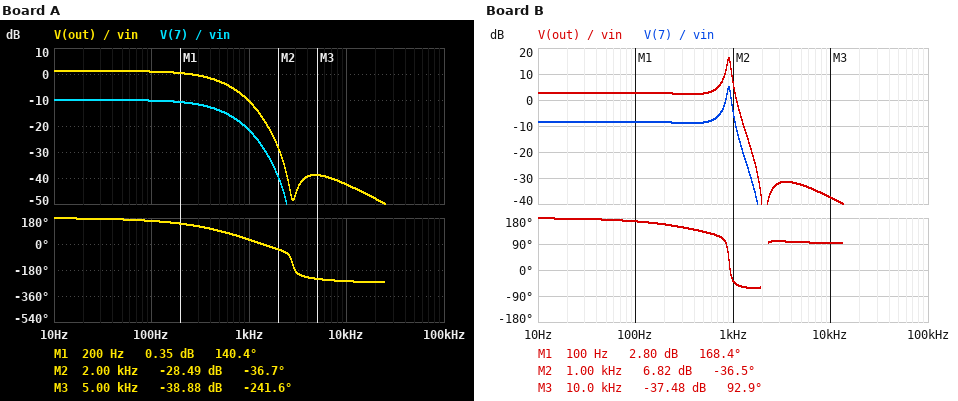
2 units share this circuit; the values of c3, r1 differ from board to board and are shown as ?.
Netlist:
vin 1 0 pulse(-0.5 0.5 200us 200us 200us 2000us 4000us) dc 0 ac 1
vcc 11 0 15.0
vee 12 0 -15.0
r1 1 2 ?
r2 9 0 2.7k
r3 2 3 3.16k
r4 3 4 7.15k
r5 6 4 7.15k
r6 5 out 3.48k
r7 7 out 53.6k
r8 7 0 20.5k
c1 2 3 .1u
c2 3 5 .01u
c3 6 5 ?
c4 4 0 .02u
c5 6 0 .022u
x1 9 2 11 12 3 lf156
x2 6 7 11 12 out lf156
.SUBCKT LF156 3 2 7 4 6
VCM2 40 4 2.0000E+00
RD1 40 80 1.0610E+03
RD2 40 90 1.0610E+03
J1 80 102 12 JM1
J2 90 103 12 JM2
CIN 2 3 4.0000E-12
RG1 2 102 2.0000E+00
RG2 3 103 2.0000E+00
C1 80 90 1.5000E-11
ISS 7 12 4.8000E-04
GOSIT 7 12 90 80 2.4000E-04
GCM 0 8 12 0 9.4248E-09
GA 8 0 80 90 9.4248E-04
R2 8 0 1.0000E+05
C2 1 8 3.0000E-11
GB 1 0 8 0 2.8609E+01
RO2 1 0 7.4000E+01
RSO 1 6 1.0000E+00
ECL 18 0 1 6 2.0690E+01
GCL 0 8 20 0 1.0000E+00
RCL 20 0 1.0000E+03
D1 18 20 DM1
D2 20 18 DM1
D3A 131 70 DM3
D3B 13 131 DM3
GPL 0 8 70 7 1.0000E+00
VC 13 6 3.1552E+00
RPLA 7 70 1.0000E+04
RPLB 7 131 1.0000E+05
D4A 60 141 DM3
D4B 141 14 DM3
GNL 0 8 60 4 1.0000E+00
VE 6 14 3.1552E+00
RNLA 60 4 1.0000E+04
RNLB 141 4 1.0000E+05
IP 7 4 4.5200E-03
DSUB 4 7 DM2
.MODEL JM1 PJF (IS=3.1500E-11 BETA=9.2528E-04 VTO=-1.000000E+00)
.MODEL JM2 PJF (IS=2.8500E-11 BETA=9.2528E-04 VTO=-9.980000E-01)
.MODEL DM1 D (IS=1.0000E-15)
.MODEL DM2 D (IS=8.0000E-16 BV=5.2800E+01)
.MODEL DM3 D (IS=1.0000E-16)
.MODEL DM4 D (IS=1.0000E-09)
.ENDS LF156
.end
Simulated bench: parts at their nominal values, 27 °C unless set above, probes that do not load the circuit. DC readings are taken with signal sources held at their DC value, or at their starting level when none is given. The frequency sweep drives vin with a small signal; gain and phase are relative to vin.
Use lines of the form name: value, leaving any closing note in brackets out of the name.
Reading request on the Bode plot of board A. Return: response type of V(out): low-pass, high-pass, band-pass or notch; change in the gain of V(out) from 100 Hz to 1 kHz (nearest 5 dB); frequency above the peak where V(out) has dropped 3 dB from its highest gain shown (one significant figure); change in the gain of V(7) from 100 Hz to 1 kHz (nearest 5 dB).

response type of V(out): low-pass, high-pass, band-pass or notch: low-pass
change in the gain of V(out) from 100 Hz to 1 kHz: -10 dB
frequency above the peak where V(out) has dropped 3 dB from its highest gain shown: 400 Hz
change in the gain of V(7) from 100 Hz to 1 kHz: -10 dB
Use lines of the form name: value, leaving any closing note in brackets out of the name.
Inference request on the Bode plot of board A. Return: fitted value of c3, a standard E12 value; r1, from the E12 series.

fitted value of c3, a standard E12 value: 5.6 nF
r1, from the E12 series: 10 kΩ
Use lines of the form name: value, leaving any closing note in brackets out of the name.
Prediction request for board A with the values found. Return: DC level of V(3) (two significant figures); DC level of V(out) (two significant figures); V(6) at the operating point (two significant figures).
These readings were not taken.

DC level of V(3): 2.6 mV
DC level of V(out): 17 mV
V(6) at the operating point: 2.6 mV
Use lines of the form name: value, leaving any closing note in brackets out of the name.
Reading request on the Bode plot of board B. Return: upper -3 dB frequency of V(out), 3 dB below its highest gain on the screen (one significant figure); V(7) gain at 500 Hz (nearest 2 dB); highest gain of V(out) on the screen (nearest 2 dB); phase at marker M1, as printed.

upper -3 dB frequency of V(out), 3 dB below its highest gain on the screen: 900 Hz
V(7) gain at 500 Hz: -8 dB
highest gain of V(out) on the screen: 16 dB
phase at marker M1, as printed: 168.4 deg
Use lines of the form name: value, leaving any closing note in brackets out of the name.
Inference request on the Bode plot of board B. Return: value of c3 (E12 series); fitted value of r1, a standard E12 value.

value of c3: 12 nF
fitted value of r1, a standard E12 value: 8.2 kΩ
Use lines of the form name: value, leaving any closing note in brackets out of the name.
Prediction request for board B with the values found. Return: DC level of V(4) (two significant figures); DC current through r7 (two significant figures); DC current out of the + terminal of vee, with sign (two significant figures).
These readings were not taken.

DC level of V(4): 2.8 mV
DC current through r7: 230 nA
DC current out of the + terminal of vee, with sign: -10 mA
